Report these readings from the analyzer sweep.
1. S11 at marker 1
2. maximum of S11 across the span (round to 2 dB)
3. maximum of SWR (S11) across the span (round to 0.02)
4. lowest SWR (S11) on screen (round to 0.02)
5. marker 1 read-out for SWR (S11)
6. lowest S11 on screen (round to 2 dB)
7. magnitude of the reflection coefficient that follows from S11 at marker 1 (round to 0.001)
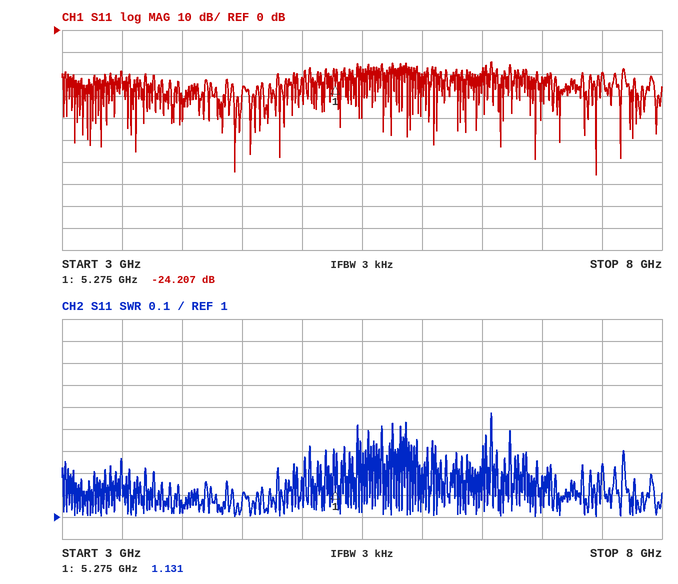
-24.207 dB
-14 dB
1.48
1.00
1.131
-66 dB
0.062
